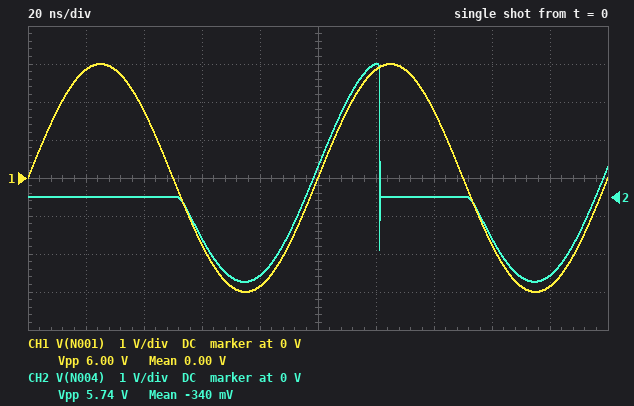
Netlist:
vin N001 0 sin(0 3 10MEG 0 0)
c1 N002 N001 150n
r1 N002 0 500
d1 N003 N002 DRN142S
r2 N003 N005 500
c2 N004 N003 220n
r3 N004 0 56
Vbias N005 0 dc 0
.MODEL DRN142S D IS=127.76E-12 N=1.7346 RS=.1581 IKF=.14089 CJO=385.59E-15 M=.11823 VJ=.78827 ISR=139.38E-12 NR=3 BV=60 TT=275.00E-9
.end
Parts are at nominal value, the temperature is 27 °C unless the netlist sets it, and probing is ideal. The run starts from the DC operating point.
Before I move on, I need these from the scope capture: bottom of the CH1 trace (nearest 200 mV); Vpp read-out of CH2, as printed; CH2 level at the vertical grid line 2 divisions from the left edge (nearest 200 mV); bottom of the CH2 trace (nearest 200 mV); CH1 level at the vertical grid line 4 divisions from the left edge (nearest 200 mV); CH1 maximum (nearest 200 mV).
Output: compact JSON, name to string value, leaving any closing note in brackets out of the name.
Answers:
{"bottom of the CH1 trace": "-3.0 V", "Vpp read-out of CH2, as printed": "5.74 V", "CH2 level at the vertical grid line 2 divisions from the left edge": "0 V", "bottom of the CH2 trace": "-2.2 V", "CH1 level at the vertical grid line 4 divisions from the left edge": "-2.8 V", "CH1 maximum": "3.0 V"}
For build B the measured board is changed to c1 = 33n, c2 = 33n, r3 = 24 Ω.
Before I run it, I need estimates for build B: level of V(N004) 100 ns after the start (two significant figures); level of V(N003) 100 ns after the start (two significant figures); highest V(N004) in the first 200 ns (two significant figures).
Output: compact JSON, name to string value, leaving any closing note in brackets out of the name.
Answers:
{"level of V(N004) 100 ns after the start": "950 mV", "level of V(N003) 100 ns after the start": "880 mV", "highest V(N004) in the first 200 ns": "3.4 V"}
